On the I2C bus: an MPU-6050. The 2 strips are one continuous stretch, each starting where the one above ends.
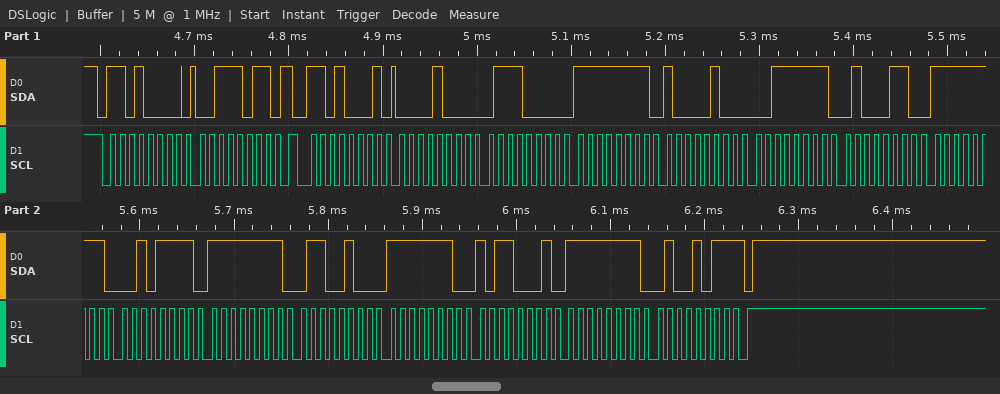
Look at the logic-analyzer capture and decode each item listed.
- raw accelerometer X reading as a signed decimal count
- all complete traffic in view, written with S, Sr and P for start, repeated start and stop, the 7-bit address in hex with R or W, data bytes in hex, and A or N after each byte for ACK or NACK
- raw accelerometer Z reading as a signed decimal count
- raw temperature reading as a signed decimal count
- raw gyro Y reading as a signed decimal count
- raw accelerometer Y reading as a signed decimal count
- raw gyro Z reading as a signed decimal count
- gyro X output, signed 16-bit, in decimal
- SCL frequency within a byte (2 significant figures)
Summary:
2160
S 68W A 3B A Sr 68R A 08 A 70 A FF A 84 A 3F A 46 A FF A 2F A FF A 64 A FE A B1 A FF A 4B N P
16198
-209
-335
-124
-181
-156
100 kHz
